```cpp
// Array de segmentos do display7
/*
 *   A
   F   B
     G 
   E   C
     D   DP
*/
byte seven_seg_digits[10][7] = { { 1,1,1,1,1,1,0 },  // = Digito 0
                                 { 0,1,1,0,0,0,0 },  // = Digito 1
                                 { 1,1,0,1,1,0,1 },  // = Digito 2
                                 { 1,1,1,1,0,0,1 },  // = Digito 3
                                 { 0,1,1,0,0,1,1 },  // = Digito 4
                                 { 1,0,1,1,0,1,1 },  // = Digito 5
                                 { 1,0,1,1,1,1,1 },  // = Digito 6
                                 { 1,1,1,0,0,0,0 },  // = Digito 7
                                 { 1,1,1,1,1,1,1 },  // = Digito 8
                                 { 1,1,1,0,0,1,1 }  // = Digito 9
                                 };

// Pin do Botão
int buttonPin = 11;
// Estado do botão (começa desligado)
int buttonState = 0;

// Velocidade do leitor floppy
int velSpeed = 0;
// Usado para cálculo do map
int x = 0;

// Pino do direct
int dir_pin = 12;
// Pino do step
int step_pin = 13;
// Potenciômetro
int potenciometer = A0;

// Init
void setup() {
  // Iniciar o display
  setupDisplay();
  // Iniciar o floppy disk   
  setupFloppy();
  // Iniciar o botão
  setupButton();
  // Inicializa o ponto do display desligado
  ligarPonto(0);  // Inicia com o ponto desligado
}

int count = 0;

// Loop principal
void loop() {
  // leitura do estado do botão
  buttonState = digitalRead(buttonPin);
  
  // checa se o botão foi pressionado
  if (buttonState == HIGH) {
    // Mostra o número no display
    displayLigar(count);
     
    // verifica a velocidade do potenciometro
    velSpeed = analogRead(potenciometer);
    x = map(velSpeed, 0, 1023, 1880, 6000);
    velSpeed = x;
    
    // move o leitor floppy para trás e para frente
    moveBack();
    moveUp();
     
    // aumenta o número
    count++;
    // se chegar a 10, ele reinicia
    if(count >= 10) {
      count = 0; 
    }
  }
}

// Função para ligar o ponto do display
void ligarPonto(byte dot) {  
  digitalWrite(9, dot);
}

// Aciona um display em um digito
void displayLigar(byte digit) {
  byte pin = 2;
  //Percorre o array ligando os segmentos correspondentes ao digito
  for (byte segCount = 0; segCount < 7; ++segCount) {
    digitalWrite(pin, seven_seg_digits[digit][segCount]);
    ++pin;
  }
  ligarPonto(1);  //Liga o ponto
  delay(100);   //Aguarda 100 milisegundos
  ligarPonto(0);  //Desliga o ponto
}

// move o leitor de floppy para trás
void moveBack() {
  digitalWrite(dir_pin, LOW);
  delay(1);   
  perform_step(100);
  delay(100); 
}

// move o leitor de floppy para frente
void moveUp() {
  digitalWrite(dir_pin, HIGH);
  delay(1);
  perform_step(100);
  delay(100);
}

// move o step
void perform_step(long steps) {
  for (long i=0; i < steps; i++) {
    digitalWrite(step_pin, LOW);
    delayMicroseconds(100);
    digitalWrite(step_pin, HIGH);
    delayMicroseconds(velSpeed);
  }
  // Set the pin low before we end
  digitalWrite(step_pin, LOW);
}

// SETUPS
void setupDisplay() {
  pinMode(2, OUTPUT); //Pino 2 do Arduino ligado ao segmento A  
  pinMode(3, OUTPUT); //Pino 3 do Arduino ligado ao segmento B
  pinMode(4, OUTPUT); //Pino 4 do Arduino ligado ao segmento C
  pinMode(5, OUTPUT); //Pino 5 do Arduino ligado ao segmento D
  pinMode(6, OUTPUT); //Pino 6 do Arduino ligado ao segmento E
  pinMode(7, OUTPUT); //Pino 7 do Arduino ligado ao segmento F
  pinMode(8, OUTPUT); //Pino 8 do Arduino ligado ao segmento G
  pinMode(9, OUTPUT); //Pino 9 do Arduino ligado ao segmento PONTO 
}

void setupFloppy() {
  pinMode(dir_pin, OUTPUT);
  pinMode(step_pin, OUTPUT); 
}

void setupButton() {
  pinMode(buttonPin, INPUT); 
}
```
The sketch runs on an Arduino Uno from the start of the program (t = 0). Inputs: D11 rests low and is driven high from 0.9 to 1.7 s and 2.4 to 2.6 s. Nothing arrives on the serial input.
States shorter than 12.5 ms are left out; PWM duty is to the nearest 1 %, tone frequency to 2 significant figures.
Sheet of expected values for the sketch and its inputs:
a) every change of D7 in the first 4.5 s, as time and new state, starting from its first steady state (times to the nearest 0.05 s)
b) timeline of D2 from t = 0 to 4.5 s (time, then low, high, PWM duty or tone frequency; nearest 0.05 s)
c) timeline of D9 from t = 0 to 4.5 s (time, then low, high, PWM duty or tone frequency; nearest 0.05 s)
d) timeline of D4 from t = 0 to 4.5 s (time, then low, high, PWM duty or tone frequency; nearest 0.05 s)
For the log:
0 s low; 0.9 s high; 1.6 s low
0 s low; 0.9 s high; 1.6 s low; 2.4 s high
0 s low; 0.9 s high; 1 s low; 1.6 s high; 1.7 s low; 2.4 s high; 2.5 s low
0 s low; 0.9 s high; 2.4 s low
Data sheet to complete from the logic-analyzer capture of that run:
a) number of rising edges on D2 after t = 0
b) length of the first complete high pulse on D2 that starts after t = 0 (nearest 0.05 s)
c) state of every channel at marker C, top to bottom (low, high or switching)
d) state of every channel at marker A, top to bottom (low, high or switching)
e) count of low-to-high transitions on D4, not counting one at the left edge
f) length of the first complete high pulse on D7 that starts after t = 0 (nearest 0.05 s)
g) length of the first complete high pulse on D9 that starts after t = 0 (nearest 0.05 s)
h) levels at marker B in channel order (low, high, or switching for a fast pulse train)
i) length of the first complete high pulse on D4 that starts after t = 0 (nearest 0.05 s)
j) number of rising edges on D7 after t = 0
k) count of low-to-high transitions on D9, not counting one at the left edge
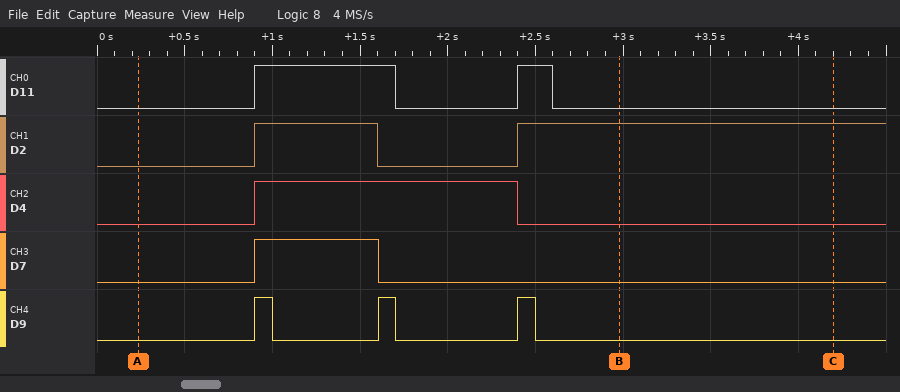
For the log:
2
0.70 s
D11 low, D2 high, D4 low, D7 low, D9 low
D11 low, D2 low, D4 low, D7 low, D9 low
1
0.70 s
0.10 s
D11 low, D2 high, D4 low, D7 low, D9 low
1.50 s
1
3
